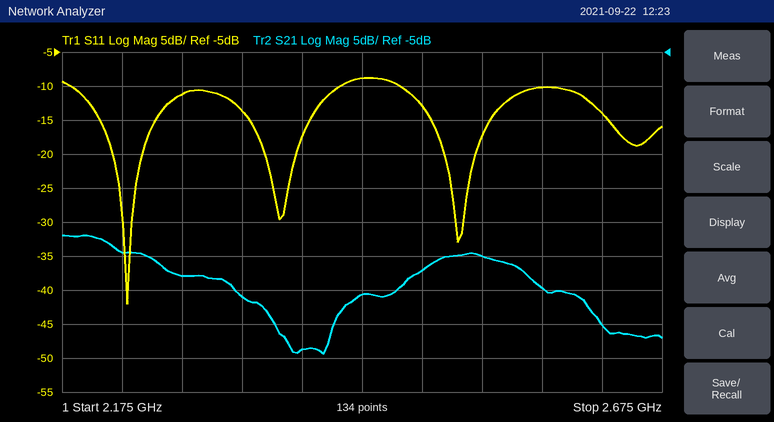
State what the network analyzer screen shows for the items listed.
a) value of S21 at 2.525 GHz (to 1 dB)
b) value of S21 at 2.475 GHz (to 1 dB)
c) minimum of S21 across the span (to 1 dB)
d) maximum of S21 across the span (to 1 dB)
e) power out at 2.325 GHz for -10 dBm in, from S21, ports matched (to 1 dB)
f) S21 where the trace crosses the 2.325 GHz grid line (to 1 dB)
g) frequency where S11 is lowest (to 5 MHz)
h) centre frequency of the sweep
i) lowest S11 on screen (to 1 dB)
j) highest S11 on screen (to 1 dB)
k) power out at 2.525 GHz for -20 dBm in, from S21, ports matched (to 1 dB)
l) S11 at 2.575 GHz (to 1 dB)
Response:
-35 dB
-37 dB
-49 dB
-32 dB
-51 dBm
-41 dB
2.230 GHz
2.425 GHz
-42 dB
-9 dB
-55 dBm
-10 dB
